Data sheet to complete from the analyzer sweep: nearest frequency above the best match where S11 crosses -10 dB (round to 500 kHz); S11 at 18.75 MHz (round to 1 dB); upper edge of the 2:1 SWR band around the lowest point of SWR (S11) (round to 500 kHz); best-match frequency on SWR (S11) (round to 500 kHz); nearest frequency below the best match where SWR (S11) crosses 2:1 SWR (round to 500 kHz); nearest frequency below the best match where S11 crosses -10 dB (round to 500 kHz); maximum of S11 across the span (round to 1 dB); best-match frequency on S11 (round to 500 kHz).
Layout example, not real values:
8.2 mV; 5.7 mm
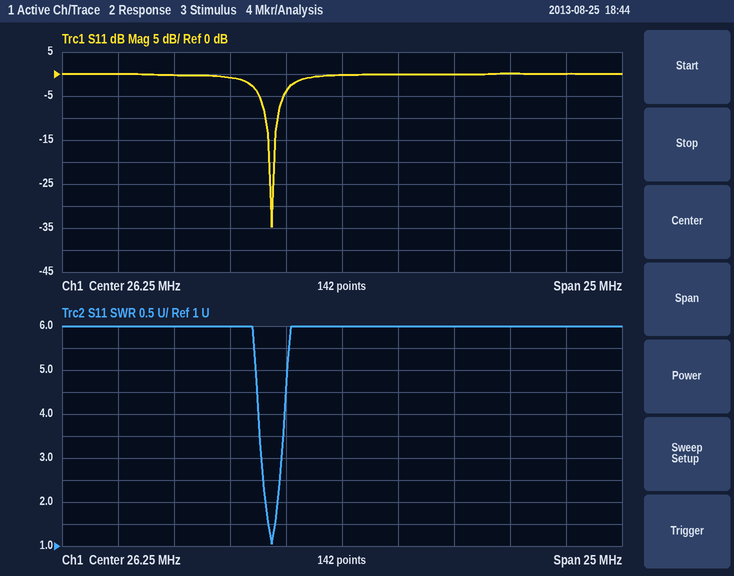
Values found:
23.5 MHz; 0 dB; 23.5 MHz; 23.0 MHz; 23.0 MHz; 23.0 MHz; 0 dB; 23.0 MHz
